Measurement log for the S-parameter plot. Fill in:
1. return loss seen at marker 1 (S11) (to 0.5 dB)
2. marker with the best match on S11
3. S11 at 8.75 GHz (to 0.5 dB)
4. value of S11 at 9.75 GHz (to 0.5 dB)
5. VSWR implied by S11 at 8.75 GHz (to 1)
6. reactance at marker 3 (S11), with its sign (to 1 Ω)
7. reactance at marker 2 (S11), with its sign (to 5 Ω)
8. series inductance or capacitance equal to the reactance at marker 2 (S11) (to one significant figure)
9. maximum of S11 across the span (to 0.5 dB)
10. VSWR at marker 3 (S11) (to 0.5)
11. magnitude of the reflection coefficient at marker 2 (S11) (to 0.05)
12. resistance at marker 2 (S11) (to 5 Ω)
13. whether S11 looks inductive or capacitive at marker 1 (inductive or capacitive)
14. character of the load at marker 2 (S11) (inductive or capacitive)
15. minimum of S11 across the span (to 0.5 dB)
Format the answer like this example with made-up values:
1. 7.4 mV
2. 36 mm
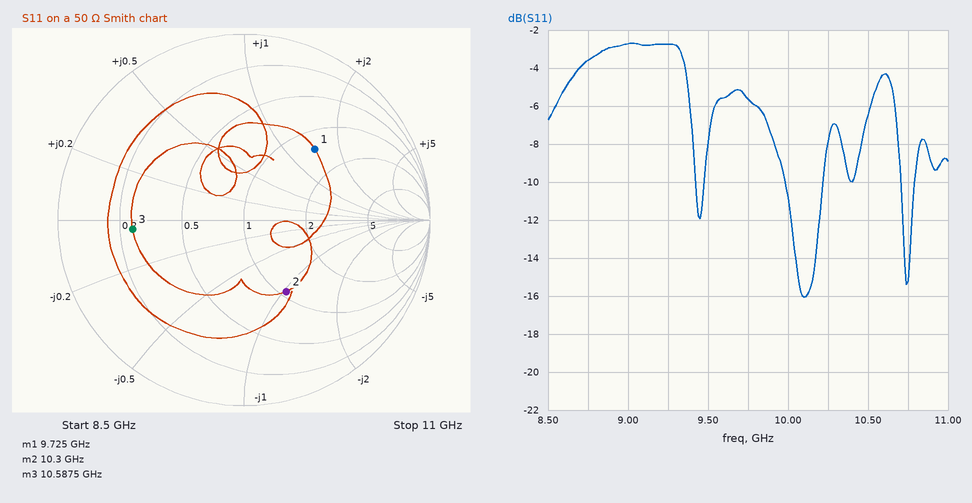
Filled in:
1. 5.5 dB
2. marker 2
3. -3.5 dB
4. -5.5 dB
5. 5
6. -2 Ω
7. -50 Ω
8. 300 fF
9. -2.5 dB
10. 4.0
11. 0.45
12. 55 Ω
13. inductive
14. capacitive
15. -16.0 dB
